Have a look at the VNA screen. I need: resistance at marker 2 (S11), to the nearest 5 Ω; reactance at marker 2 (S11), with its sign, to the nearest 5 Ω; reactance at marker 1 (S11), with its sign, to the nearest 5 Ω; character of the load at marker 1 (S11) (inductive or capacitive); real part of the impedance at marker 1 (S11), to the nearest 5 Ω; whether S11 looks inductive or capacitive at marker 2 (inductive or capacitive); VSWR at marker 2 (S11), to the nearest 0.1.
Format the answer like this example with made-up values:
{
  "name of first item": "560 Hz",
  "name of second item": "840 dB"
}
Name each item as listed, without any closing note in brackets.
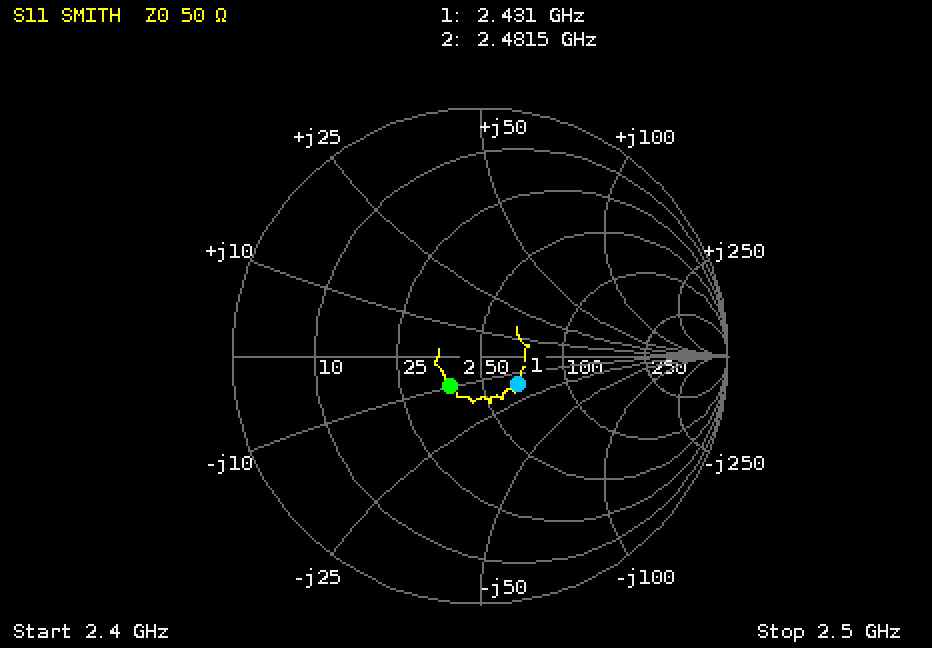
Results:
{
  "resistance at marker 2 (S11), to the nearest 5 Ω": "40 Ω",
  "reactance at marker 2 (S11), with its sign, to the nearest 5 Ω": "-10 Ω",
  "reactance at marker 1 (S11), with its sign, to the nearest 5 Ω": "-15 Ω",
  "character of the load at marker 1 (S11)": "capacitive",
  "real part of the impedance at marker 1 (S11), to the nearest 5 Ω": "65 Ω",
  "whether S11 looks inductive or capacitive at marker 2": "capacitive",
  "VSWR at marker 2 (S11), to the nearest 0.1": "1.4"
}
